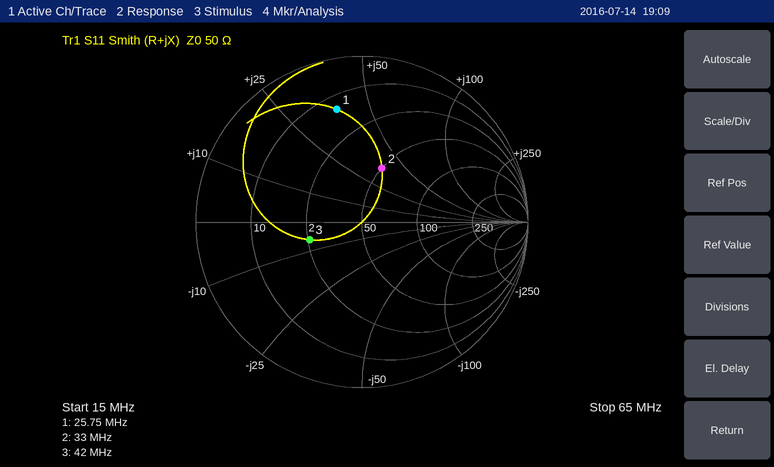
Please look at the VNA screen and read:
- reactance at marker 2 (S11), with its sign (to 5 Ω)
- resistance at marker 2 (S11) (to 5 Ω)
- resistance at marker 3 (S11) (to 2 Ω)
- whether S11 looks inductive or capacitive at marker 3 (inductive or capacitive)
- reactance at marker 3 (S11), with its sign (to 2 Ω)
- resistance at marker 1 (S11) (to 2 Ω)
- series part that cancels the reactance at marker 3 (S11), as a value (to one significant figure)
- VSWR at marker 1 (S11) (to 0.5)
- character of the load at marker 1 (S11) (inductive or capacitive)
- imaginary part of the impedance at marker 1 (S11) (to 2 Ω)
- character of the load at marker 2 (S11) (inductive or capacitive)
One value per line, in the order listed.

+35 Ω
50 Ω
26 Ω
capacitive
-6 Ω
14 Ω
20 nH
5.5
inductive
+38 Ω
inductive
